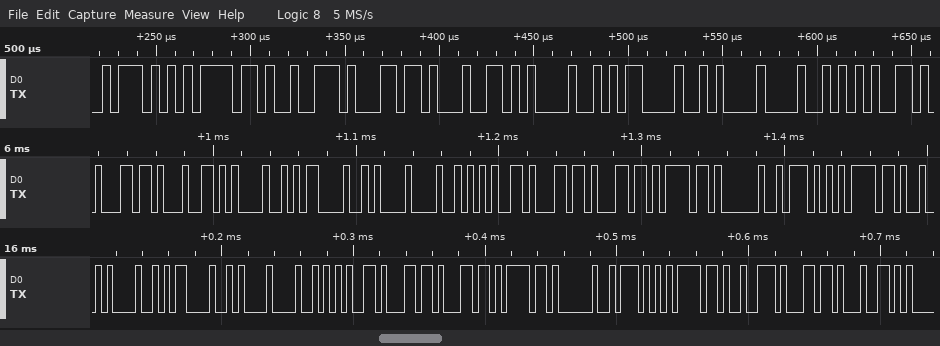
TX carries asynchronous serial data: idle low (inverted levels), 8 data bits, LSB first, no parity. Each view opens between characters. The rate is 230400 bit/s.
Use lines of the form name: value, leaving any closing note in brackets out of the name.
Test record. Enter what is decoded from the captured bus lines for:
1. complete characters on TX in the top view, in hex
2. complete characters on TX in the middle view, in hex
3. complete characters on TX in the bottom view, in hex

complete characters on TX in the top view, in hex: 51, 21, 1B, 27, 37, BD, E5, EB, 6F, 35
complete characters on TX in the middle view, in hex: 27, 37, BD, E5, EB, 6F, 35, 27, 27, 21, BF, 51, 21
complete characters on TX in the bottom view, in hex: BD, E5, EB, 6F, 35, 27, 27, 21, BF, 51, 21, 1B, 27, 37
